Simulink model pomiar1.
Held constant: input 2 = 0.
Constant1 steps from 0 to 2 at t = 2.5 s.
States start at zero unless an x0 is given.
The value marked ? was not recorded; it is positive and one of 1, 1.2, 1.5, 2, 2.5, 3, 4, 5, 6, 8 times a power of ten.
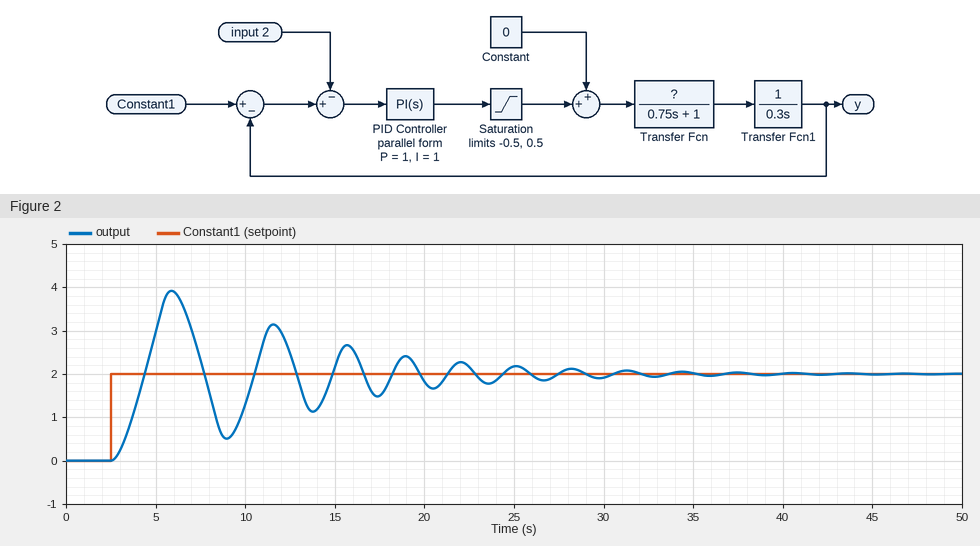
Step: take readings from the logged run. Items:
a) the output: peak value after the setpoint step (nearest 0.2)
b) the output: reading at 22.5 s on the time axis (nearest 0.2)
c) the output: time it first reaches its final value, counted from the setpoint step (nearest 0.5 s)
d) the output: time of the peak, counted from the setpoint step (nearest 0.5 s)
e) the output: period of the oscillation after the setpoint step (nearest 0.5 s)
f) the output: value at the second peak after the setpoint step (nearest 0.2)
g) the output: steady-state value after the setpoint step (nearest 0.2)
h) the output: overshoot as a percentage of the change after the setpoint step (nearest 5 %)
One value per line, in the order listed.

4.0
2.2
2.0 s
3.5 s
5.5 s
3.2
2.0
95 %
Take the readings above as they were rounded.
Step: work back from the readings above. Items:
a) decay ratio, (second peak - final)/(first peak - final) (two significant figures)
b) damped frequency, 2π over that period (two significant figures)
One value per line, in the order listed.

0.60
1.1 rad/s
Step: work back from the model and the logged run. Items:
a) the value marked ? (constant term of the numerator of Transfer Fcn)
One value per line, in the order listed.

1
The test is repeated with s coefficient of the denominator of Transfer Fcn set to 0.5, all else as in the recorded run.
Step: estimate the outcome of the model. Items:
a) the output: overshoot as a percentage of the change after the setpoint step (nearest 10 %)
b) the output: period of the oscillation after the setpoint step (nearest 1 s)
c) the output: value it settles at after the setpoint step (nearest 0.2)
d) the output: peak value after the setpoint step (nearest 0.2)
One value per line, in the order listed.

80 %
4 s
2.0
3.6
